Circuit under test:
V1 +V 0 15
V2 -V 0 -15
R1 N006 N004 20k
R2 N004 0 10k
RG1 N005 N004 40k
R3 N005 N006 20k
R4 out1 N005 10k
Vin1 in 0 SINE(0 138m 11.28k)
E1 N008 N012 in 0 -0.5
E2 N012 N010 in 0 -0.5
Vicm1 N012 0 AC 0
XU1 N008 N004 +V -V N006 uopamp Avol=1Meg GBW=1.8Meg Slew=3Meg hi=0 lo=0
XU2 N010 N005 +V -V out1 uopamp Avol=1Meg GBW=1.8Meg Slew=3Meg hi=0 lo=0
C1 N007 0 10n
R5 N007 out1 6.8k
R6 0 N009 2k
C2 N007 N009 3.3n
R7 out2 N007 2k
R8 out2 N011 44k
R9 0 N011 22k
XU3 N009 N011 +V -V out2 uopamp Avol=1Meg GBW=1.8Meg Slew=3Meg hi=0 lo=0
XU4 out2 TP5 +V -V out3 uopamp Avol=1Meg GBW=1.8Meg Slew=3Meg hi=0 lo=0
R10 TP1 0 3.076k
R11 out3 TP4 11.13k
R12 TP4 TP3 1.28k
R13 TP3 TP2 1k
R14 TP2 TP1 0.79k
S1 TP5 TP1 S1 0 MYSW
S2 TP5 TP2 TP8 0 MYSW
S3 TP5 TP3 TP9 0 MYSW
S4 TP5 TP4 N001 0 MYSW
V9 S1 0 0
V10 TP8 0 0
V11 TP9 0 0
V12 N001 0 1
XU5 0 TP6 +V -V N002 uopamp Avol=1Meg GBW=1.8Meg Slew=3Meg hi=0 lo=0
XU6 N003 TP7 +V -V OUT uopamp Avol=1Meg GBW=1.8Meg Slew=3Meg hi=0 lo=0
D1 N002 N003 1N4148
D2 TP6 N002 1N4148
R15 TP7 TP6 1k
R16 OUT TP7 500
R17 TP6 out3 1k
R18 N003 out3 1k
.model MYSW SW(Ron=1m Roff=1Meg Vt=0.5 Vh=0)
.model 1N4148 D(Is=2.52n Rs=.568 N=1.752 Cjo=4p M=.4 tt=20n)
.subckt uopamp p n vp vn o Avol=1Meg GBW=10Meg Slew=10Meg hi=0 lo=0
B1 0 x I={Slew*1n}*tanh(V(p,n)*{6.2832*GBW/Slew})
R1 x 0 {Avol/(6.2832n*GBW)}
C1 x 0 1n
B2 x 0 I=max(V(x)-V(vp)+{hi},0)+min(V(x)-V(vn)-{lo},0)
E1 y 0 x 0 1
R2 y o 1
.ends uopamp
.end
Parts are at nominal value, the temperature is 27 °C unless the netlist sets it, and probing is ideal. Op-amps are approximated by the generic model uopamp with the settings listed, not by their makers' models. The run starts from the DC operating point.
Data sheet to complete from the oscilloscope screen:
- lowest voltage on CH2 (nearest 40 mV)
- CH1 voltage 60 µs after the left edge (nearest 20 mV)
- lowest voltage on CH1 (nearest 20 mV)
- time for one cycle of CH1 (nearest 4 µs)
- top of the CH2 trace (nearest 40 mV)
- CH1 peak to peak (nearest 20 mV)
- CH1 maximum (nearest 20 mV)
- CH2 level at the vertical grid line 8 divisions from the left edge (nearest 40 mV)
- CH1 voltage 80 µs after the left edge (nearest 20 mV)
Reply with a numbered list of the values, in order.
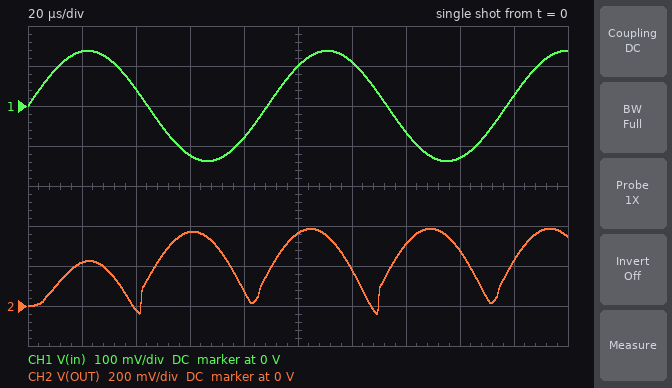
1. -40 mV
2. -120 mV
3. -140 mV
4. 88 µs
5. 400 mV
6. 280 mV
7. 140 mV
8. 280 mV
9. -80 mV
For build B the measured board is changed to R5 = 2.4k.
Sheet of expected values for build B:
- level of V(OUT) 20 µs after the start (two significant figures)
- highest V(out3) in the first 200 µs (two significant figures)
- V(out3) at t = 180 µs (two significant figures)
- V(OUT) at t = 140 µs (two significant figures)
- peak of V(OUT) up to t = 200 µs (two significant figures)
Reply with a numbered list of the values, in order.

1. 490 mV
2. 520 mV
3. 380 mV
4. 700 mV
5. 770 mV
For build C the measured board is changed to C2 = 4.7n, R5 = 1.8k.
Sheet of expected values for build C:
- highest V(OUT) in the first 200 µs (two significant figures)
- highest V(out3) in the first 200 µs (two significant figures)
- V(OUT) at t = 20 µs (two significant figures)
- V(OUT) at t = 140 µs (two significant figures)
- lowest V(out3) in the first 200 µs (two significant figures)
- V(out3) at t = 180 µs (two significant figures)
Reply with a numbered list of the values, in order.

1. 1.4 V
2. 920 mV
3. 800 mV
4. 1.2 V
5. -920 mV
6. 650 mV
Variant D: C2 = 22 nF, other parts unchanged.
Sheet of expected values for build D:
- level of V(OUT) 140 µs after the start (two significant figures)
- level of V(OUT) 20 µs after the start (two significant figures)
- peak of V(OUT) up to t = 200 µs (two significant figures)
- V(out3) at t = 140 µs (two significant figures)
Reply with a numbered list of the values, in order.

1. 1.3 V
2. 560 mV
3. 2.6 V
4. 870 mV
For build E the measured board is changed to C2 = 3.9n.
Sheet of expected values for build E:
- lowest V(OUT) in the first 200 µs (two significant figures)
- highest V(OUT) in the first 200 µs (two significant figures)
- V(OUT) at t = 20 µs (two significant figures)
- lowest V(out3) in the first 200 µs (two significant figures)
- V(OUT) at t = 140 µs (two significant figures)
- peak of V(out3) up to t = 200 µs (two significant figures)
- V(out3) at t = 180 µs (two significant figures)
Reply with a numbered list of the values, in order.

1. -47 mV
2. 500 mV
3. 250 mV
4. -330 mV
5. 380 mV
6. 330 mV
7. 180 mV
